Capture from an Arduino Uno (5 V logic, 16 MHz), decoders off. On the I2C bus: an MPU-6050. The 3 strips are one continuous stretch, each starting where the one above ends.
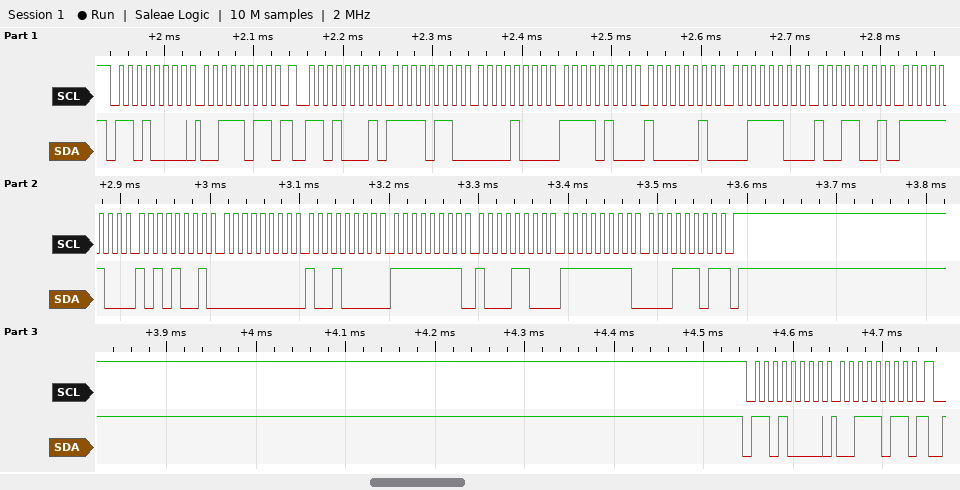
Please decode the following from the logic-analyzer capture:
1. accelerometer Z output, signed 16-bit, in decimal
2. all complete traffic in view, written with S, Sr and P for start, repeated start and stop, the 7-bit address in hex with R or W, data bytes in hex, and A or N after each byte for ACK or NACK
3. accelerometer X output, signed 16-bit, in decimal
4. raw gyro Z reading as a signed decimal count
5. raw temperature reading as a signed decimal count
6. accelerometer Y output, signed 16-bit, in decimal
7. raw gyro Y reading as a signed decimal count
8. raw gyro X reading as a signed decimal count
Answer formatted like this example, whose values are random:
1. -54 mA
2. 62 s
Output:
1. 15513
2. S 68W A 3B A Sr 68R A F6 A 08 A F4 A 82 A 3C A 99 A FC A A9 A 00 A 90 A FF A 8C A FF A 1D N P S 68W A 3B A
3. -2552
4. -227
5. -855
6. -2942
7. -116
8. 144
